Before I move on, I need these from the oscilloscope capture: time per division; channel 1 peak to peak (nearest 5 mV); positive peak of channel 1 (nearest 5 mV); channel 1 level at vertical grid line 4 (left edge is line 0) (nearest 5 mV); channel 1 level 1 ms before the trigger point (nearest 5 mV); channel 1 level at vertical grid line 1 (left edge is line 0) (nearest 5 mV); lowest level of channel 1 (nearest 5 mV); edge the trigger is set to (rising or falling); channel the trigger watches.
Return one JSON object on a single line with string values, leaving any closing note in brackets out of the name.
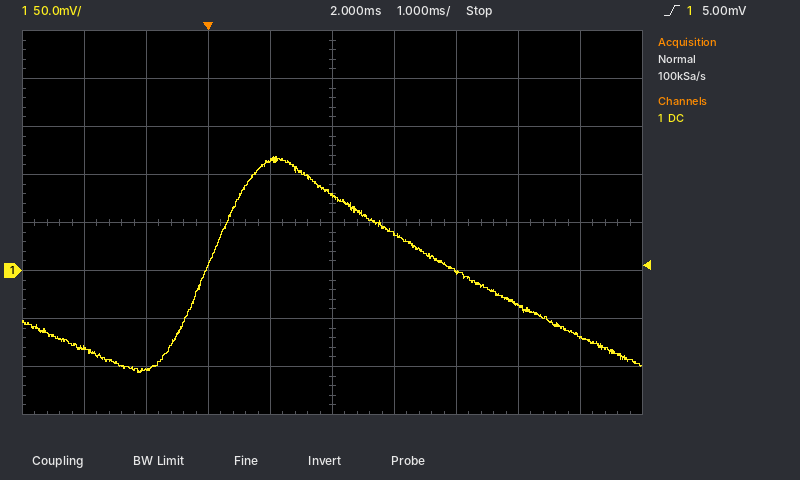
{"time per division": "1 ms", "channel 1 peak to peak": "225 mV", "positive peak of channel 1": "120 mV", "channel 1 level at vertical grid line 4 (left edge is line 0)": "115 mV", "channel 1 level 1 ms before the trigger point": "-105 mV", "channel 1 level at vertical grid line 1 (left edge is line 0)": "-80 mV", "lowest level of channel 1": "-105 mV", "edge the trigger is set to": "rising", "channel the trigger watches": "channel 1"}
